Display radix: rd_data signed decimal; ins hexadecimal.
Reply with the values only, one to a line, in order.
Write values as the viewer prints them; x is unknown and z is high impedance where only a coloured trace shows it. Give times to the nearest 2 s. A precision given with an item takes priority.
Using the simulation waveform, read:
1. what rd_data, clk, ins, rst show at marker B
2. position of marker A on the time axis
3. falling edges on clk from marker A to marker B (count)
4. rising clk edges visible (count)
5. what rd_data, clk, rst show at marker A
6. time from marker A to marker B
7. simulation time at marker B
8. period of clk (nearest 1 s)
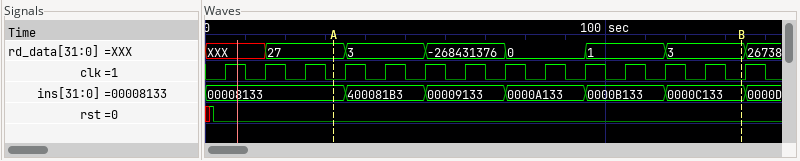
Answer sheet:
rd_data=3, clk=0, ins=0000C133, rst=0
32 s
10
14
rd_data=27, clk=0, rst=0
102 s
134 s
10 s
